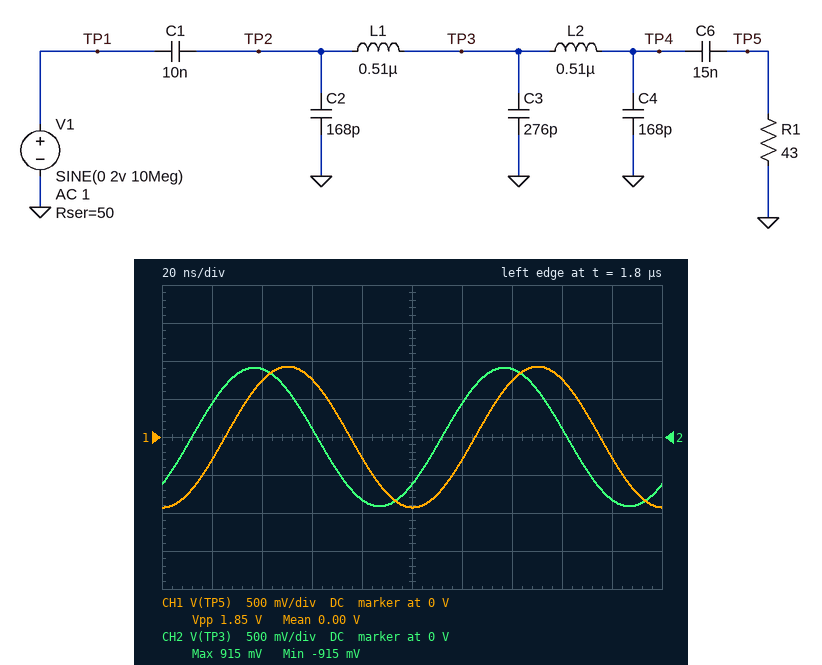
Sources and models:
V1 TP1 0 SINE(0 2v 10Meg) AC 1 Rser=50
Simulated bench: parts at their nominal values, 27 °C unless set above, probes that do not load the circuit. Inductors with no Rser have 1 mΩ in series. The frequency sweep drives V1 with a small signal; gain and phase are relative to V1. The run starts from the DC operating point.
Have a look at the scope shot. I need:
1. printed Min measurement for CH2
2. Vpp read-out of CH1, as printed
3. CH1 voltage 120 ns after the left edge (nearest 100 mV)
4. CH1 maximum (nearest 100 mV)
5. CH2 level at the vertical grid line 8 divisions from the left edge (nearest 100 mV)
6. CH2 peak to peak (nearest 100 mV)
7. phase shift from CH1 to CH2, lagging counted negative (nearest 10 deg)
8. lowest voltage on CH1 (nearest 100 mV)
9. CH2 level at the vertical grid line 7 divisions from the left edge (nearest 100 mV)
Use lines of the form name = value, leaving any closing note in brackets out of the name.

printed Min measurement for CH2 = -915 mV
Vpp read-out of CH1, as printed = 1.85 V
CH1 voltage 120 ns after the left edge = -300 mV
CH1 maximum = 900 mV
CH2 level at the vertical grid line 8 divisions from the left edge = 100 mV
CH2 peak to peak = 1.8 V
phase shift from CH1 to CH2, lagging counted negative = 50 deg
lowest voltage on CH1 = -900 mV
CH2 level at the vertical grid line 7 divisions from the left edge = 900 mV
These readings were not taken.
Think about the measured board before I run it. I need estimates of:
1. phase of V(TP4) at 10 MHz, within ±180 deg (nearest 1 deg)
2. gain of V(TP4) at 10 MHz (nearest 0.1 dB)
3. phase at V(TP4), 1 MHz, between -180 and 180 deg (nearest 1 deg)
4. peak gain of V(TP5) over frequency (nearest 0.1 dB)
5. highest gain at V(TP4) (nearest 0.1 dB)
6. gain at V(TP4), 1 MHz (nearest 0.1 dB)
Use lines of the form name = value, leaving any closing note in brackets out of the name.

phase of V(TP4) at 10 MHz, within ±180 deg = -92 deg
gain of V(TP4) at 10 MHz = -6.7 dB
phase at V(TP4), 1 MHz, between -180 and 180 deg = -7 deg
peak gain of V(TP5) over frequency = -6.7 dB
highest gain at V(TP4) = -6.7 dB
gain at V(TP4), 1 MHz = -6.8 dB
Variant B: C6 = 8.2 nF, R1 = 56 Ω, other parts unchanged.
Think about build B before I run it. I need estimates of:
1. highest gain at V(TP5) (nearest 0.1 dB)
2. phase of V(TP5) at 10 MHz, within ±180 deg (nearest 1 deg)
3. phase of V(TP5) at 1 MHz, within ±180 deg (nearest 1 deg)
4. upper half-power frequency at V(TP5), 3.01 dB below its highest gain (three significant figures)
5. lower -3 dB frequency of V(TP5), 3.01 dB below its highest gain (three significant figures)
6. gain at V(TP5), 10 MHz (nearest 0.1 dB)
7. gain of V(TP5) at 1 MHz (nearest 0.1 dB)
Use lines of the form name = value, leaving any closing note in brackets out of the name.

highest gain at V(TP5) = -5.5 dB
phase of V(TP5) at 10 MHz, within ±180 deg = -90 deg
phase of V(TP5) at 1 MHz, within ±180 deg = 10 deg
upper half-power frequency at V(TP5), 3.01 dB below its highest gain = 25.0 MHz
lower -3 dB frequency of V(TP5), 3.01 dB below its highest gain = 350 kHz
gain at V(TP5), 10 MHz = -5.6 dB
gain of V(TP5) at 1 MHz = -6.1 dB
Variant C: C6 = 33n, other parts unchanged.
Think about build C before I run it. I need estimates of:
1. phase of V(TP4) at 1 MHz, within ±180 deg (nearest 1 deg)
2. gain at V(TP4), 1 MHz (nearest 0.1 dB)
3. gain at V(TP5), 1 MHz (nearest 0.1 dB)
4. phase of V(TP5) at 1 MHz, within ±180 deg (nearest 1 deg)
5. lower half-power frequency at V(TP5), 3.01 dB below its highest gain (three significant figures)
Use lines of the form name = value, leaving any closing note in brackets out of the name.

phase of V(TP4) at 1 MHz, within ±180 deg = -3 deg
gain at V(TP4), 1 MHz = -6.9 dB
gain at V(TP5), 1 MHz = -6.9 dB
phase of V(TP5) at 1 MHz, within ±180 deg = 4 deg
lower half-power frequency at V(TP5), 3.01 dB below its highest gain = 228 kHz
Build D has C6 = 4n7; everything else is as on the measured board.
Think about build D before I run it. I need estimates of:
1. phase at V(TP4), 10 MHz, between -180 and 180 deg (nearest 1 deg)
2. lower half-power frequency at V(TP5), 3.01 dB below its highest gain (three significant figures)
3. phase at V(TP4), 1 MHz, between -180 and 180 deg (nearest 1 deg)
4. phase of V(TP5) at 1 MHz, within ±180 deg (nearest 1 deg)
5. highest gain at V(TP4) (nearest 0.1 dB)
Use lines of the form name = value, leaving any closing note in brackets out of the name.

phase at V(TP4), 10 MHz, between -180 and 180 deg = -94 deg
lower half-power frequency at V(TP5), 3.01 dB below its highest gain = 567 kHz
phase at V(TP4), 1 MHz, between -180 and 180 deg = -18 deg
phase of V(TP5) at 1 MHz, within ±180 deg = 20 deg
highest gain at V(TP4) = -3.7 dB
